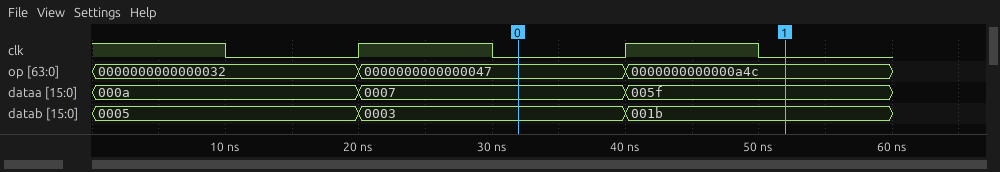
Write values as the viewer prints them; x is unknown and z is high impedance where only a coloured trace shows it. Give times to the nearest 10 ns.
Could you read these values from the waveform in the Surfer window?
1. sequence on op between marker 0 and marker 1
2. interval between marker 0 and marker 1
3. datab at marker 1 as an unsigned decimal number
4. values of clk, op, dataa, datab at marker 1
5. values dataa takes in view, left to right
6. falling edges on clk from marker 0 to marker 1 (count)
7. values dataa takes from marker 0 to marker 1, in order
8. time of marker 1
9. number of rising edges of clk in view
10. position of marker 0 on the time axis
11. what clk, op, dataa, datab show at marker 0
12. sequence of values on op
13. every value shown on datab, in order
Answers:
0000000000000047, 0000000000000a4c
20 ns
27
clk=0, op=0000000000000a4c, dataa=005f, datab=001b
000a, 0007, 005f
1
0007, 005f
50 ns
2
30 ns
clk=0, op=0000000000000047, dataa=0007, datab=0003
0000000000000032, 0000000000000047, 0000000000000a4c
0005, 0003, 001b
